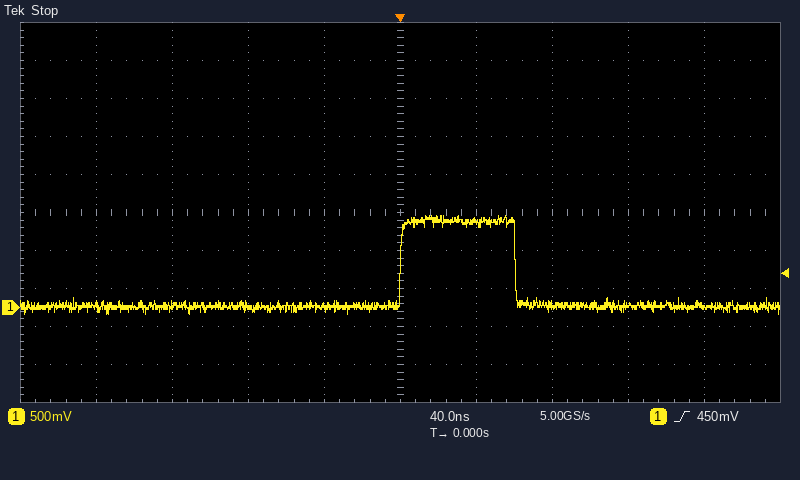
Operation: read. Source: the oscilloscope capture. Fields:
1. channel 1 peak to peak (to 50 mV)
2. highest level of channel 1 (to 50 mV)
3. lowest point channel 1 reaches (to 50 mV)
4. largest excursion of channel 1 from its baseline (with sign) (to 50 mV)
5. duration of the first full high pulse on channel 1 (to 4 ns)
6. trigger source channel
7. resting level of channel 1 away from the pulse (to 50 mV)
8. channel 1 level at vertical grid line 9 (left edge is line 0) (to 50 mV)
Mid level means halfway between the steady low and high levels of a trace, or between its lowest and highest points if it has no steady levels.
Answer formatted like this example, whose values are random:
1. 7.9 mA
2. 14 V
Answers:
1. 1.30 V
2. 1.20 V
3. -100 mV
4. +1.20 V
5. 60 ns
6. channel 1
7. 0 mV
8. 0 mV
